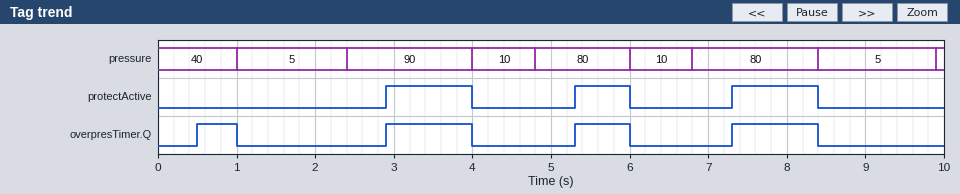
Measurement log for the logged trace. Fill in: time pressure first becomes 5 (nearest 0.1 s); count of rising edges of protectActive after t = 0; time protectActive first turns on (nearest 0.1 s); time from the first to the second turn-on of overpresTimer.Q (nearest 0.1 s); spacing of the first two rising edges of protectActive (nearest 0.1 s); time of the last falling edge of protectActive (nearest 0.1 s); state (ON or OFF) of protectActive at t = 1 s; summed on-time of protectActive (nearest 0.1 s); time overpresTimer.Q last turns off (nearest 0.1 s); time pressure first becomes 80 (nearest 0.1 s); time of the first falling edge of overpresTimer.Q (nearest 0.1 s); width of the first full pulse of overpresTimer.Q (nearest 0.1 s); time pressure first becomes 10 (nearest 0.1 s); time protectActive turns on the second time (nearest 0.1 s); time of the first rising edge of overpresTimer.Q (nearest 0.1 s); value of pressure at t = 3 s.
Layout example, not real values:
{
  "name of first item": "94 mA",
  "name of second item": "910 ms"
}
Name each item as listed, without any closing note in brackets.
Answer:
{
  "time pressure first becomes 5": "1.0 s",
  "count of rising edges of protectActive after t = 0": "3",
  "time protectActive first turns on": "2.9 s",
  "time from the first to the second turn-on of overpresTimer.Q": "2.4 s",
  "spacing of the first two rising edges of protectActive": "2.4 s",
  "time of the last falling edge of protectActive": "8.4 s",
  "state (ON or OFF) of protectActive at t = 1 s": "OFF",
  "summed on-time of protectActive": "2.9 s",
  "time overpresTimer.Q last turns off": "8.4 s",
  "time pressure first becomes 80": "4.8 s",
  "time of the first falling edge of overpresTimer.Q": "1.0 s",
  "width of the first full pulse of overpresTimer.Q": "0.5 s",
  "time pressure first becomes 10": "4.0 s",
  "time protectActive turns on the second time": "5.3 s",
  "time of the first rising edge of overpresTimer.Q": "0.5 s",
  "value of pressure at t = 3 s": "90"
}
